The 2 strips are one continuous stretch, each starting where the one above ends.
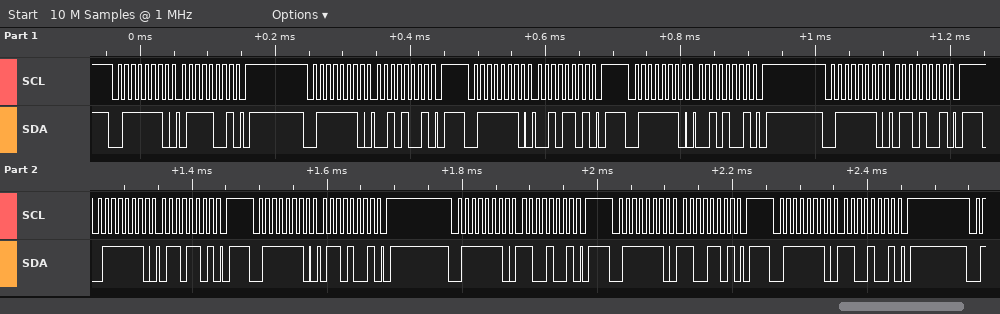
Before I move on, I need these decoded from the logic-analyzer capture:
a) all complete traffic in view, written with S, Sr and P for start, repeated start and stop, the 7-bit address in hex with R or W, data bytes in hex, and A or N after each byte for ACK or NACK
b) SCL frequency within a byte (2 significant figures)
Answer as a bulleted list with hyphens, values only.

- S 3FW A 79 A P S 3FW A 29 A P S 3FW A 2D A P S 3FW A 29 A P S 3FW A 69 A P S 3FW A 6D A P S 3FW A 69 A P S 3FW A C9 A P S 3FW A CD A P S 3FW A C9 A P
- 100 kHz
